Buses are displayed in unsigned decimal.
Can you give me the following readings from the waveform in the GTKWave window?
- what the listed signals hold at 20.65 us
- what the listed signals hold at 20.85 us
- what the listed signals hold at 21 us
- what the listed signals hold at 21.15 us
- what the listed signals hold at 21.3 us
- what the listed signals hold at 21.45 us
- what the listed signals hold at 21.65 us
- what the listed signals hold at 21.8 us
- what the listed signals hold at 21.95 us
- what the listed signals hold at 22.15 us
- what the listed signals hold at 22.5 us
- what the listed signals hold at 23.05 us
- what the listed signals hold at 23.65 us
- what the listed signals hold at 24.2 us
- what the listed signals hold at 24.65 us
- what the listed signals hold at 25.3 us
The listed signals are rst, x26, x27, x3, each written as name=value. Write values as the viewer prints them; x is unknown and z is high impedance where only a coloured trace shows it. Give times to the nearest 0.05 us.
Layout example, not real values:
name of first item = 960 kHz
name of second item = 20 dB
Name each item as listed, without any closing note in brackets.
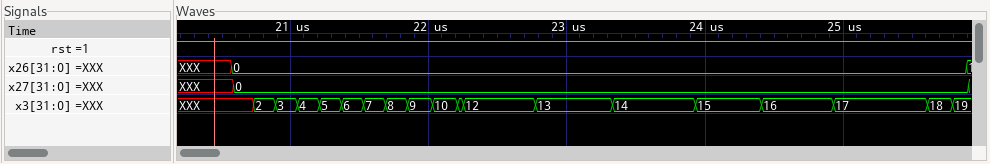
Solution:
what the listed signals hold at 20.65 us = rst=1, x26=0, x27=0, x3=XXX
what the listed signals hold at 20.85 us = rst=1, x26=0, x27=0, x3=2
what the listed signals hold at 21 us = rst=1, x26=0, x27=0, x3=3
what the listed signals hold at 21.15 us = rst=1, x26=0, x27=0, x3=4
what the listed signals hold at 21.3 us = rst=1, x26=0, x27=0, x3=5
what the listed signals hold at 21.45 us = rst=1, x26=0, x27=0, x3=6
what the listed signals hold at 21.65 us = rst=1, x26=0, x27=0, x3=7
what the listed signals hold at 21.8 us = rst=1, x26=0, x27=0, x3=8
what the listed signals hold at 21.95 us = rst=1, x26=0, x27=0, x3=9
what the listed signals hold at 22.15 us = rst=1, x26=0, x27=0, x3=10
what the listed signals hold at 22.5 us = rst=1, x26=0, x27=0, x3=12
what the listed signals hold at 23.05 us = rst=1, x26=0, x27=0, x3=13
what the listed signals hold at 23.65 us = rst=1, x26=0, x27=0, x3=14
what the listed signals hold at 24.2 us = rst=1, x26=0, x27=0, x3=15
what the listed signals hold at 24.65 us = rst=1, x26=0, x27=0, x3=16
what the listed signals hold at 25.3 us = rst=1, x26=0, x27=0, x3=17
